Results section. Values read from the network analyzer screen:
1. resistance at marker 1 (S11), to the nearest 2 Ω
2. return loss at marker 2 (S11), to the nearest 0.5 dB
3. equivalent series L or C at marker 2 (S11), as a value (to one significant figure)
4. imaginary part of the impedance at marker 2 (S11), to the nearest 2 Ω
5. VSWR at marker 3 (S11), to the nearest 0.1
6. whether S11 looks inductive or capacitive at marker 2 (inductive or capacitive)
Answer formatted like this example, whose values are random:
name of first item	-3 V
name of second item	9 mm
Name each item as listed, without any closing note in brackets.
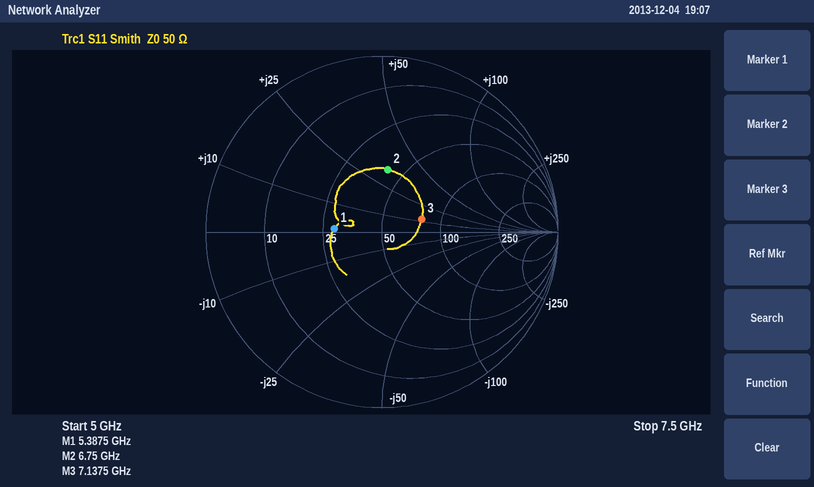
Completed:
resistance at marker 1 (S11), to the nearest 2 Ω	28 Ω
return loss at marker 2 (S11), to the nearest 0.5 dB	9.0 dB
equivalent series L or C at marker 2 (S11), as a value	800 pH
imaginary part of the impedance at marker 2 (S11), to the nearest 2 Ω	+34 Ω
VSWR at marker 3 (S11), to the nearest 0.1	1.6
whether S11 looks inductive or capacitive at marker 2	inductive
